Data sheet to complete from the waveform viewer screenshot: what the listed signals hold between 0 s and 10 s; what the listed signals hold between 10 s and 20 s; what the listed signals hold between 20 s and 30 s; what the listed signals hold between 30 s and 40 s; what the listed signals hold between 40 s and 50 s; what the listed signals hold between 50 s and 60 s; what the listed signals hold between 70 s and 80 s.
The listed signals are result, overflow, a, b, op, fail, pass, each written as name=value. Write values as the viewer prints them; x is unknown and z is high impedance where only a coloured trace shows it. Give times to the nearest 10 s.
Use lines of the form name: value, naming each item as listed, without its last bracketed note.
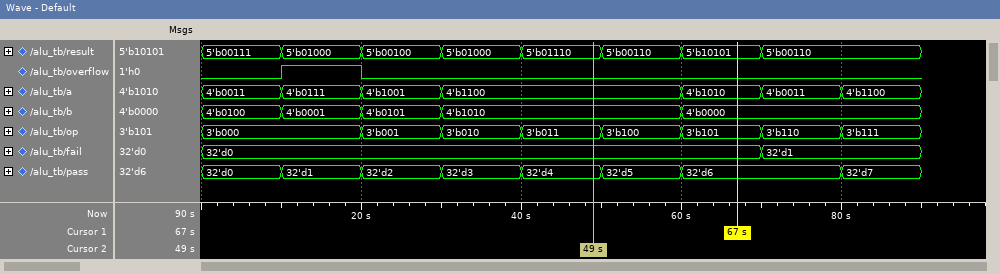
what the listed signals hold between 0 s and 10 s: result=5'b00111, overflow=0, a=4'b0011, b=4'b0100, op=3'b000, fail=32'd0, pass=32'd0
what the listed signals hold between 10 s and 20 s: result=5'b01000, overflow=1, a=4'b0111, b=4'b0001, op=3'b000, fail=32'd0, pass=32'd1
what the listed signals hold between 20 s and 30 s: result=5'b00100, overflow=0, a=4'b1001, b=4'b0101, op=3'b001, fail=32'd0, pass=32'd2
what the listed signals hold between 30 s and 40 s: result=5'b01000, overflow=0, a=4'b1100, b=4'b1010, op=3'b010, fail=32'd0, pass=32'd3
what the listed signals hold between 40 s and 50 s: result=5'b01110, overflow=0, a=4'b1100, b=4'b1010, op=3'b011, fail=32'd0, pass=32'd4
what the listed signals hold between 50 s and 60 s: result=5'b00110, overflow=0, a=4'b1100, b=4'b1010, op=3'b100, fail=32'd0, pass=32'd5
what the listed signals hold between 70 s and 80 s: result=5'b00110, overflow=0, a=4'b0011, b=4'b0000, op=3'b110, fail=32'd1, pass=32'd6
